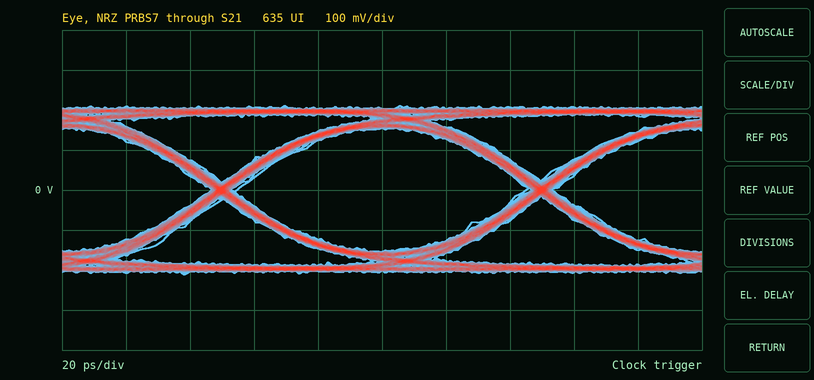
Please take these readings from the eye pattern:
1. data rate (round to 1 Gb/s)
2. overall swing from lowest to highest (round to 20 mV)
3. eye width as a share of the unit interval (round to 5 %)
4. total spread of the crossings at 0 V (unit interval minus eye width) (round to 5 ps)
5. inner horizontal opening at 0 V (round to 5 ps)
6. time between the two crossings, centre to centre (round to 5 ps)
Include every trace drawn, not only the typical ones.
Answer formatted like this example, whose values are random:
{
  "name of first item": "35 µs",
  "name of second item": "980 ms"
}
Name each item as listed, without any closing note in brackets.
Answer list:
{
  "data rate": "10 Gb/s",
  "overall swing from lowest to highest": "420 mV",
  "eye width as a share of the unit interval": "90 %",
  "total spread of the crossings at 0 V (unit interval minus eye width)": "10 ps",
  "inner horizontal opening at 0 V": "90 ps",
  "time between the two crossings, centre to centre": "100 ps"
}
